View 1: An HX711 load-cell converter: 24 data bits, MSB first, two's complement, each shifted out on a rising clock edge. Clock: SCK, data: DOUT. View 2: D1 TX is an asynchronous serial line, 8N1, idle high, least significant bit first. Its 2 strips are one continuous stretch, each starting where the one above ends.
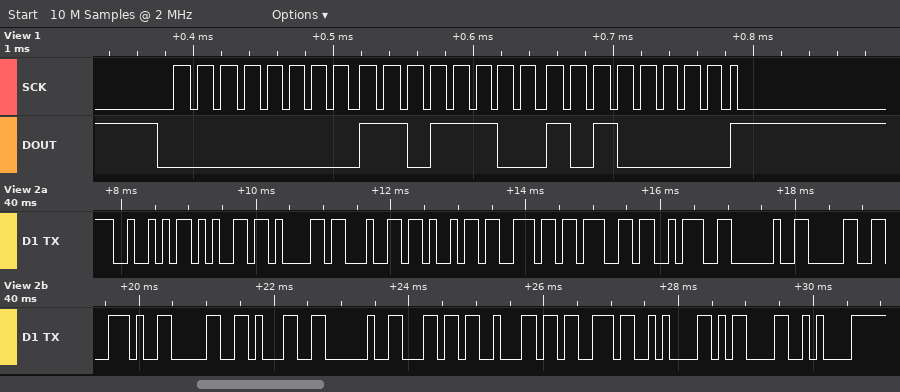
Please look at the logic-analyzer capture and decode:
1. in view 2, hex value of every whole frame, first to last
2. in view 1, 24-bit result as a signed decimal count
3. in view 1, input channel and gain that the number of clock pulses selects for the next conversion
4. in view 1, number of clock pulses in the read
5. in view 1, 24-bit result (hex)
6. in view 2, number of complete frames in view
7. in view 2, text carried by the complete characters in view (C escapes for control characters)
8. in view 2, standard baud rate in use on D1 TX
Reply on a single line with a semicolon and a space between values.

52 65 61 64 69 6E 67 3A 20 30 2E 30 31 20 6C 62 73 0A 0D 0A; 56480; channel A, gain 128; 25; 0x00DCA0; 20; "Reading: 0.01 lbs\n\r\n"; 9600 baud
